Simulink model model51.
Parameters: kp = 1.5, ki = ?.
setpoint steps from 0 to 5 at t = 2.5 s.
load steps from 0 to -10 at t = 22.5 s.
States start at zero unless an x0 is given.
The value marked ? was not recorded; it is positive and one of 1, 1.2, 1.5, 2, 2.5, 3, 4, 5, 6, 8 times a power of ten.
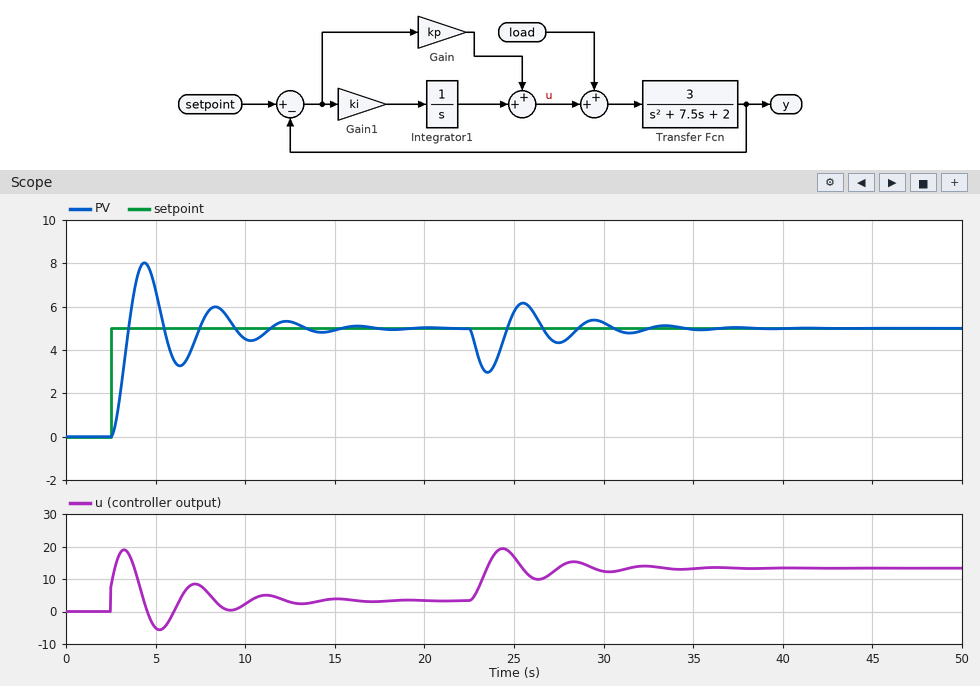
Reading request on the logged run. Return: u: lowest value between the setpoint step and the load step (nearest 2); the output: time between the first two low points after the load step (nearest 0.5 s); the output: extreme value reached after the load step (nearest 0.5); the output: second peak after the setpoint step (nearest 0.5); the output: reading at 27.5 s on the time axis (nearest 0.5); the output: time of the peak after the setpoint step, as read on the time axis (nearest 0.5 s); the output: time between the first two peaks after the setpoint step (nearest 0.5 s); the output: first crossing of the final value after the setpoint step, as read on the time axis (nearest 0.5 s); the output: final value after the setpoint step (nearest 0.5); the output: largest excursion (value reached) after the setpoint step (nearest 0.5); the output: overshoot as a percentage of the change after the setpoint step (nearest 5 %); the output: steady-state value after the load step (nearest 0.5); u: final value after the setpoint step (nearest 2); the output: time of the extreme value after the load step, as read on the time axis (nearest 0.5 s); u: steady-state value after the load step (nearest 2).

-6
4.0 s
3.0
6.0
4.5
4.5 s
4.0 s
3.5 s
5.0
8.0
60 %
5.0
4
23.5 s
14
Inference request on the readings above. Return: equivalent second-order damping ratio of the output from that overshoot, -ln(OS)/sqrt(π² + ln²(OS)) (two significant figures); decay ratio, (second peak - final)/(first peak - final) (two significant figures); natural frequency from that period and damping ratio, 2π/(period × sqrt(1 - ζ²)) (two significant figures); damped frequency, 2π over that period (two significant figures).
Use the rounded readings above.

0.16
0.33
1.6 rad/s
1.6 rad/s
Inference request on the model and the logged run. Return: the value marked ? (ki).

6
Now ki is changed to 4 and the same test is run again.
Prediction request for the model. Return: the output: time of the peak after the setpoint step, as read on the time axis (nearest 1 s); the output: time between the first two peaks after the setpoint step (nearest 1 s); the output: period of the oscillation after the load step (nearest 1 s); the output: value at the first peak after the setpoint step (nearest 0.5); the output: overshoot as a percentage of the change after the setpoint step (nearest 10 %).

5 s
5 s
5 s
7.5
50 %
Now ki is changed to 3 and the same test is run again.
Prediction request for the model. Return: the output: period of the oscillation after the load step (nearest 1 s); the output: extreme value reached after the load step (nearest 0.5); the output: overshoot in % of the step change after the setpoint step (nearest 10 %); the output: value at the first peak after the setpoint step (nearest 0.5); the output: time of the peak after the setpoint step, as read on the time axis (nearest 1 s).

6 s
2.5
40 %
7.0
5 s
